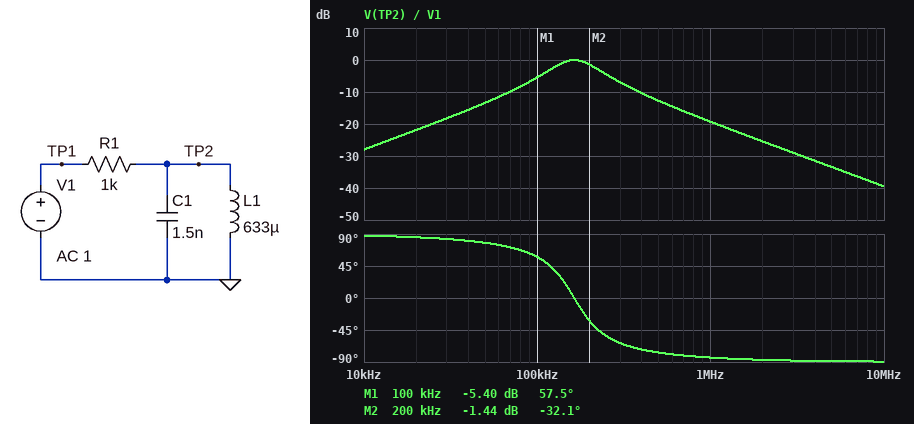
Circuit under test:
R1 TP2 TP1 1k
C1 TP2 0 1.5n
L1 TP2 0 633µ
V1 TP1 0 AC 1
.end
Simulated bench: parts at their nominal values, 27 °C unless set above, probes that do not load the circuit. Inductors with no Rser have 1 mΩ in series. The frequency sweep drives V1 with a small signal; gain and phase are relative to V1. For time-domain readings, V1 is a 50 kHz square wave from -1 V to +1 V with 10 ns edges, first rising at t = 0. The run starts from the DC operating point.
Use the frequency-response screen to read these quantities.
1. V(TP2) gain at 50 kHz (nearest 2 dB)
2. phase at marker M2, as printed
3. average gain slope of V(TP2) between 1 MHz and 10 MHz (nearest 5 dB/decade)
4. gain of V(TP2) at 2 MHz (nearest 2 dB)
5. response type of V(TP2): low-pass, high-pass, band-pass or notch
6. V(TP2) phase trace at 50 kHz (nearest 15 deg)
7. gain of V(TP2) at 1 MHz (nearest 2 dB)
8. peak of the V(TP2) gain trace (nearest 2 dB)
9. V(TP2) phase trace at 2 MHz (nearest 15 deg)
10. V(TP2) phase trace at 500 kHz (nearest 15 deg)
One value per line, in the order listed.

-14 dB
-32.1 deg
-20 dB/decade
-26 dB
band-pass
75 deg
-20 dB
0 dB
-90 deg
-75 deg
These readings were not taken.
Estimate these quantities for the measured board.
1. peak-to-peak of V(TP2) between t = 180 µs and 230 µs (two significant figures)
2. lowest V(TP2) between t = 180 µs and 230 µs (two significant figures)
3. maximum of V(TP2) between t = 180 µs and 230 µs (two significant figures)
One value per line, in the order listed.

1.8 V
-880 mV
880 mV
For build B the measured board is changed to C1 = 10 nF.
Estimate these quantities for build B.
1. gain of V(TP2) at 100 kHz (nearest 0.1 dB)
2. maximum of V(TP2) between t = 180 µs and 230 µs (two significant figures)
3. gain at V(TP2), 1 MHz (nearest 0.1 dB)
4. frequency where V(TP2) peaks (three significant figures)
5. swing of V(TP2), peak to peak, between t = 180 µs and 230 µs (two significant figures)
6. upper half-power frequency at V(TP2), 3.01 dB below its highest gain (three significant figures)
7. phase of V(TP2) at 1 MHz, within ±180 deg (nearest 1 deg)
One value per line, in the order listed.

-11.8 dB
630 mV
-35.9 dB
63.3 kHz
1.3 V
71.7 kHz
-89 deg
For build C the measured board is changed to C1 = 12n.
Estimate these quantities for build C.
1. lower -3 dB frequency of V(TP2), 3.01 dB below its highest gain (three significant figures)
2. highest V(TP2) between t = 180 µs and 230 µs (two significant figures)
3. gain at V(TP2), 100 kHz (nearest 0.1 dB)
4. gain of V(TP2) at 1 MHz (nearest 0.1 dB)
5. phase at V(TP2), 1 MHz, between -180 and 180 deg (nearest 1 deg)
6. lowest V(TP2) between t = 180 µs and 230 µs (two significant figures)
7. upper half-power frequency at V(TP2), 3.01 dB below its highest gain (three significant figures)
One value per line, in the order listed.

51.5 kHz
830 mV
-14.2 dB
-37.5 dB
-89 deg
-830 mV
64.8 kHz
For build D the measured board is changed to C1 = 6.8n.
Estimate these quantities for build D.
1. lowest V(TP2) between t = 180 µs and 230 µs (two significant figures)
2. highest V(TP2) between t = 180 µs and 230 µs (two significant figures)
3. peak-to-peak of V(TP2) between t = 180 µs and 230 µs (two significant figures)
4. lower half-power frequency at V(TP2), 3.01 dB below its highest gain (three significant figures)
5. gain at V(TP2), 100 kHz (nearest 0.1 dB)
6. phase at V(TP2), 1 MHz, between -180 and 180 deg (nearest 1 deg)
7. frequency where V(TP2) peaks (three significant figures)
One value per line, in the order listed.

-460 mV
460 mV
930 mV
65.9 kHz
-6.1 dB
-89 deg
76.7 kHz
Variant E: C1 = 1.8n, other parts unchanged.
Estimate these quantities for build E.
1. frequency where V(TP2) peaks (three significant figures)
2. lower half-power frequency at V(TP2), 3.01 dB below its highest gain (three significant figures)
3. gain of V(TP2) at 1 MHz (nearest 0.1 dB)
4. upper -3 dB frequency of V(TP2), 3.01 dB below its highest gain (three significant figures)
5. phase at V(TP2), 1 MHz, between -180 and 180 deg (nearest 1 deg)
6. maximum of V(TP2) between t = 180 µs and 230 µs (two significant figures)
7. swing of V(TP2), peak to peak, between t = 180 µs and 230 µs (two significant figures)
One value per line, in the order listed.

149 kHz
111 kHz
-20.9 dB
200 kHz
-85 deg
840 mV
1.7 V
